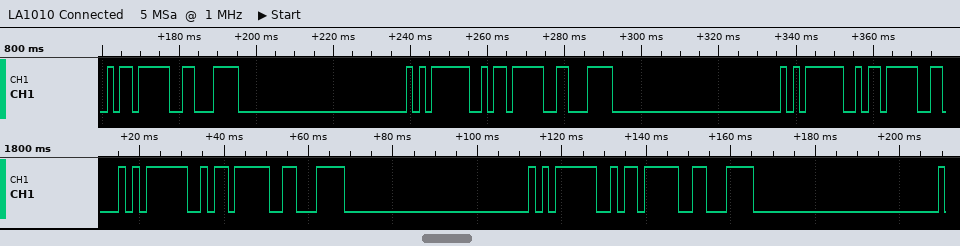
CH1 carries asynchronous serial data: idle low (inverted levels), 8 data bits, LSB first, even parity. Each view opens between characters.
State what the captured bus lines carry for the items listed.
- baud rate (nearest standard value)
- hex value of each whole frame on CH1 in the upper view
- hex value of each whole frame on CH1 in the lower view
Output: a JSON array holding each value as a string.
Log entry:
["600 baud", "09, 0E, 05, 09, 0E, 05, 09", "05, 09, 0E, 05, 09, 0E"]
